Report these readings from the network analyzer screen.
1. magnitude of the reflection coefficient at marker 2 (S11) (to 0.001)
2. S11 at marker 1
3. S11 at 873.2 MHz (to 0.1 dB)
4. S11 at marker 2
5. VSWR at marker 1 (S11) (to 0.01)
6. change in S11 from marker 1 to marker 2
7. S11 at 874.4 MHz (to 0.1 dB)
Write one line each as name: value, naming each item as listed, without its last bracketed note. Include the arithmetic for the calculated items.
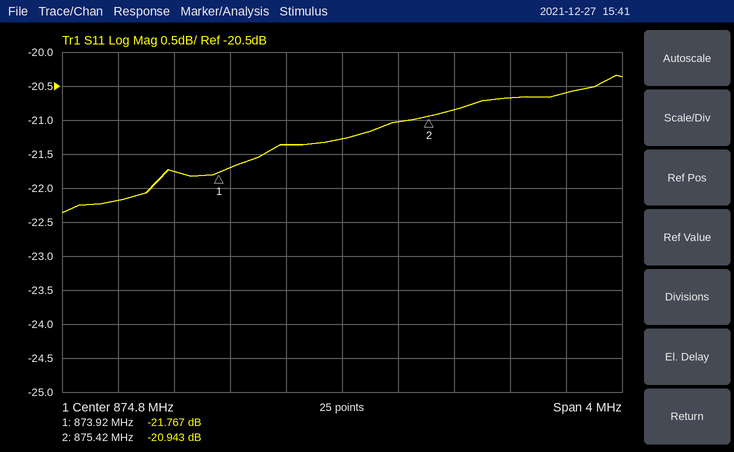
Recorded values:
magnitude of the reflection coefficient at marker 2 (S11): 10^(-20.943/20) ≈ 0.090
S11 at marker 1: -21.767 dB
S11 at 873.2 MHz: -22.2 dB
S11 at marker 2: -20.943 dB
VSWR at marker 1 (S11): (1 + 0.0816)/(1 − 0.0816) ≈ 1.18
change in S11 from marker 1 to marker 2: -20.943 − (-21.767) = 0.824 dB
S11 at 874.4 MHz: -21.4 dB
